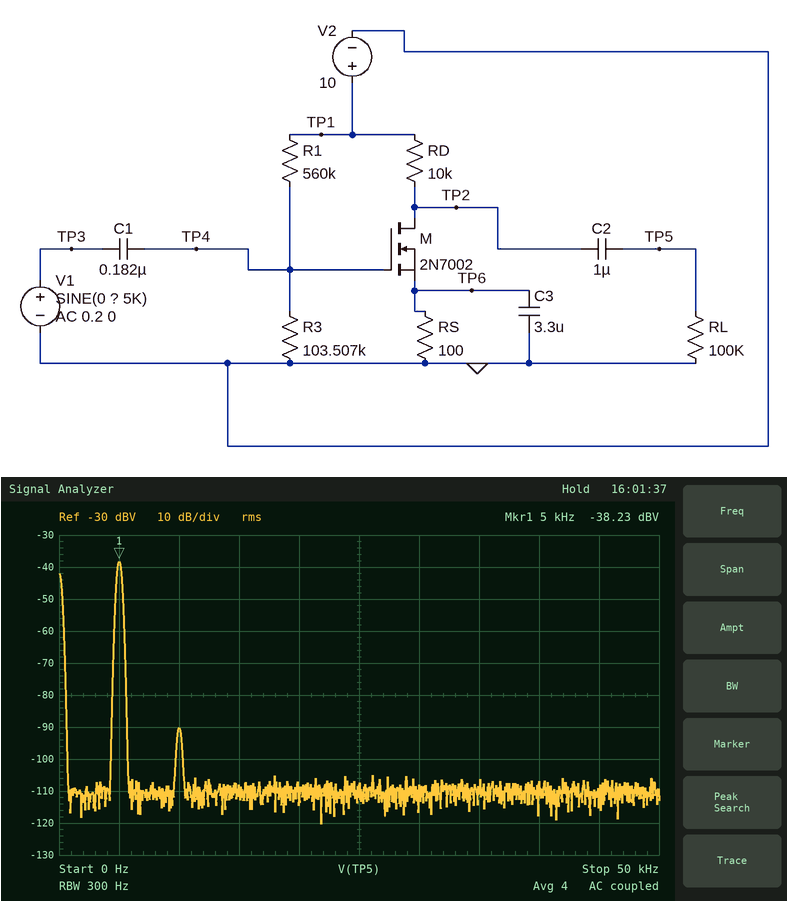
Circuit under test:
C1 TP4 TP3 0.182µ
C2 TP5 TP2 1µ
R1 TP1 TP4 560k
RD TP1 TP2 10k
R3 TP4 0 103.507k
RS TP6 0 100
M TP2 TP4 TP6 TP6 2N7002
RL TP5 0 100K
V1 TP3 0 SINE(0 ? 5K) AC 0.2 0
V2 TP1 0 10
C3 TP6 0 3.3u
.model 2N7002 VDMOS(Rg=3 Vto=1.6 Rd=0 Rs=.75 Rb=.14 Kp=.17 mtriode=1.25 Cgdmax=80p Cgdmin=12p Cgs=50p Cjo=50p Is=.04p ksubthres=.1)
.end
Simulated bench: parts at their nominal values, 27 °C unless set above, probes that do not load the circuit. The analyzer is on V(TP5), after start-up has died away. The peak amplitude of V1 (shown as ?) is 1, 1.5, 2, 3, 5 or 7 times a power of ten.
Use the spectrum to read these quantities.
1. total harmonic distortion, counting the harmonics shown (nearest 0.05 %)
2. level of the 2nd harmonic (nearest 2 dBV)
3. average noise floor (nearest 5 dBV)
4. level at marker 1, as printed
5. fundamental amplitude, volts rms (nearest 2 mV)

0.25 %
-90 dBV
-110 dBV
-38.23 dBV
12 mV
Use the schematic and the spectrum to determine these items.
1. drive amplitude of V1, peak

700 µV
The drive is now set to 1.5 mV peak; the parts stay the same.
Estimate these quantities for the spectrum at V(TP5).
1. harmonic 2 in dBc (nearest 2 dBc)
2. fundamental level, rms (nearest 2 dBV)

-46 dBc
-32 dBV
